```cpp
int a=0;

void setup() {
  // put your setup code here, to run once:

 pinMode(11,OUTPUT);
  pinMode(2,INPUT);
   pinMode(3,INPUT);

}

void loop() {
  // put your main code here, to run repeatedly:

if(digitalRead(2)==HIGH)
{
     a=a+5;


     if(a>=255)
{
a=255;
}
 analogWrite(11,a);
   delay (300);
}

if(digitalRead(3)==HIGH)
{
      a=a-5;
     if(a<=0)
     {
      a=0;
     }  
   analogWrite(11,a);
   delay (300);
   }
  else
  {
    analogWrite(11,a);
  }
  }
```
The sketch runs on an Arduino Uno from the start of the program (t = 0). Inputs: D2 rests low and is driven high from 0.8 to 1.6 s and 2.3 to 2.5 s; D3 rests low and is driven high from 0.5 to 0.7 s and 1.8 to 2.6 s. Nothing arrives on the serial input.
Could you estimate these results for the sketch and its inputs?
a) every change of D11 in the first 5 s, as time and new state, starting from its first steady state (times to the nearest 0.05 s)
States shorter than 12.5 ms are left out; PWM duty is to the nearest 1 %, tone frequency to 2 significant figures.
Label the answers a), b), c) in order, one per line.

a) 0 s low; 0.8 s PWM 2 %; 1.1 s PWM 4 %; 1.4 s PWM 6 %; 1.8 s PWM 4 %; 2.1 s PWM 2 %; 2.4 s PWM 4 %
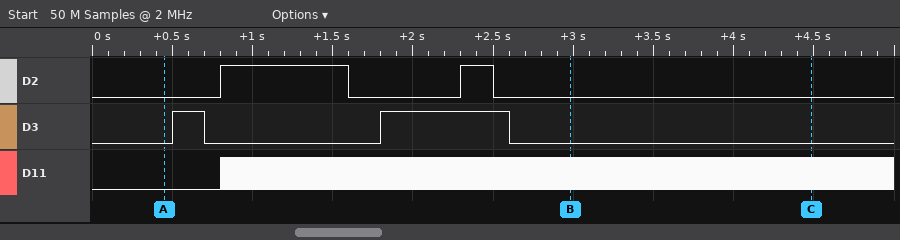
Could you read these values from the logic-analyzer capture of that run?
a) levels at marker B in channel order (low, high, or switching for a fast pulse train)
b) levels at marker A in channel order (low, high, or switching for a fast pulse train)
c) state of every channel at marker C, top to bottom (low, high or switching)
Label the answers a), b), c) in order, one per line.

a) D2 low, D3 low, D11 switching
b) D2 low, D3 low, D11 low
c) D2 low, D3 low, D11 switching
